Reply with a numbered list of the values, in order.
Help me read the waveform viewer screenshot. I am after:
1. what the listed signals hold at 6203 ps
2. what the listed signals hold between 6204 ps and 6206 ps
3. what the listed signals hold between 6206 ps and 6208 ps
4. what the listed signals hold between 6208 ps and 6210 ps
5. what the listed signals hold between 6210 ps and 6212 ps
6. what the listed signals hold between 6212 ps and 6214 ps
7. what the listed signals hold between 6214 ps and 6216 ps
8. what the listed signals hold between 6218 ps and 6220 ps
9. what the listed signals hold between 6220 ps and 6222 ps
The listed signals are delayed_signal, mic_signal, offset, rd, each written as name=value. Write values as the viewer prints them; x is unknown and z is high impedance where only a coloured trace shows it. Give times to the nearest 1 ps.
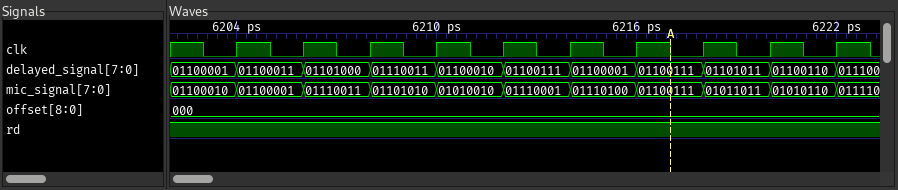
1. delayed_signal=01100001, mic_signal=01100010, offset=000, rd=1
2. delayed_signal=01100011, mic_signal=01100001, offset=000, rd=1
3. delayed_signal=01101000, mic_signal=01110011, offset=000, rd=1
4. delayed_signal=01110011, mic_signal=01101010, offset=000, rd=1
5. delayed_signal=01100010, mic_signal=01010010, offset=000, rd=1
6. delayed_signal=01100111, mic_signal=01110001, offset=000, rd=1
7. delayed_signal=01100001, mic_signal=01110100, offset=000, rd=1
8. delayed_signal=01101011, mic_signal=01011011, offset=000, rd=1
9. delayed_signal=01100110, mic_signal=01010110, offset=000, rd=1
